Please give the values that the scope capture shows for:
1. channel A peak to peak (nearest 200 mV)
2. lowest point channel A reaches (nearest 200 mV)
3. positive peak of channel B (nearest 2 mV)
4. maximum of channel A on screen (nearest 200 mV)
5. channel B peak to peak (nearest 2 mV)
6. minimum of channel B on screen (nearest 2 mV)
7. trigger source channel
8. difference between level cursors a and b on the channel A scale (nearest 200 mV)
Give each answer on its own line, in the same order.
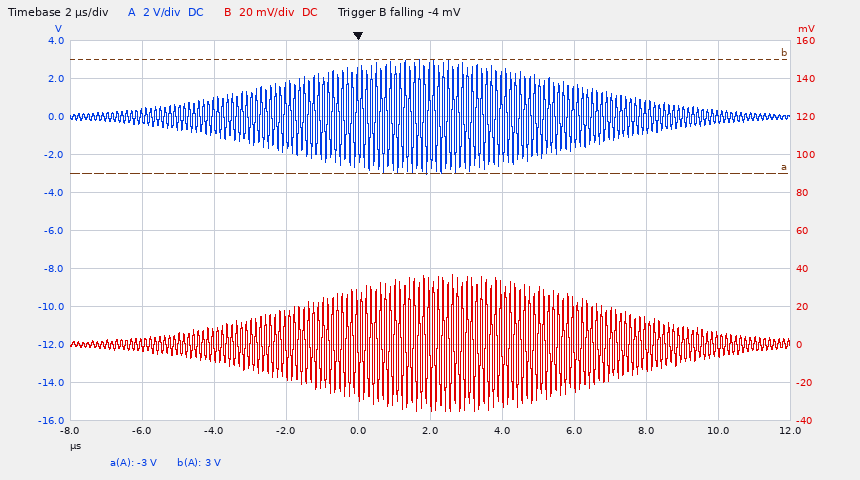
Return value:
6.0 V
-3.0 V
36 mV
3.0 V
72 mV
-36 mV
channel B
6.0 V
